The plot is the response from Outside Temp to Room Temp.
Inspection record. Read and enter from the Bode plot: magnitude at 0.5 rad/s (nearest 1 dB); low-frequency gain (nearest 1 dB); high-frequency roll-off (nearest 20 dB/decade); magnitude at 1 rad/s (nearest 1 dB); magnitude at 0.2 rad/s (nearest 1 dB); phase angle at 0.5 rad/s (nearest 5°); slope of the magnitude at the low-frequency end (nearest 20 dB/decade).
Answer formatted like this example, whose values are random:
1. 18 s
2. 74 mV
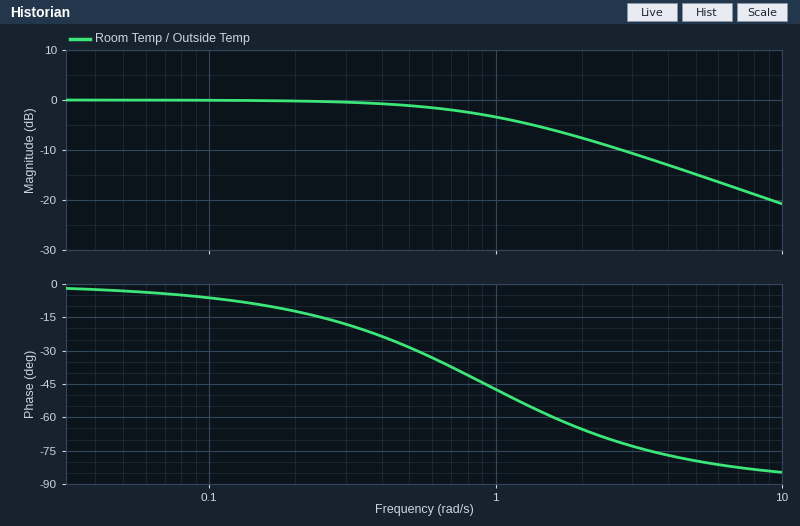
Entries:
1. -1 dB
2. 0 dB
3. -20 dB/decade
4. -3 dB
5. 0 dB
6. -30°
7. 0 dB/decade
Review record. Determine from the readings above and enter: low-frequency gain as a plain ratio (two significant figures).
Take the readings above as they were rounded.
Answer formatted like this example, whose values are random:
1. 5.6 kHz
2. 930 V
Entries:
1. 1.0
